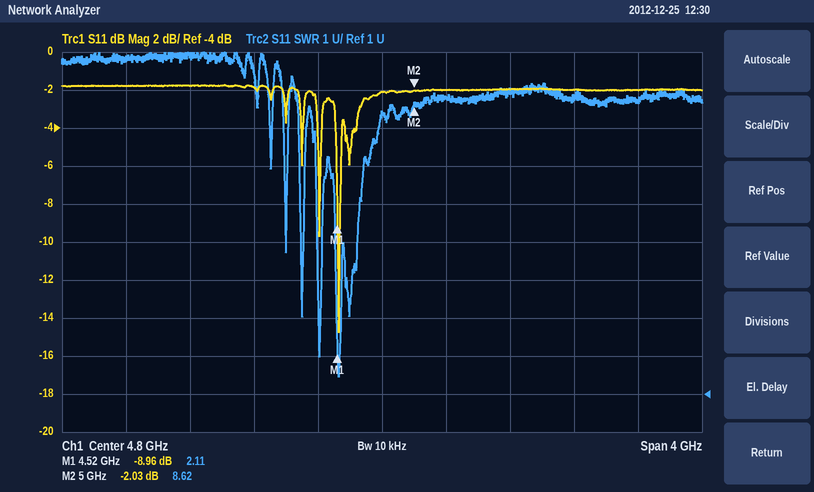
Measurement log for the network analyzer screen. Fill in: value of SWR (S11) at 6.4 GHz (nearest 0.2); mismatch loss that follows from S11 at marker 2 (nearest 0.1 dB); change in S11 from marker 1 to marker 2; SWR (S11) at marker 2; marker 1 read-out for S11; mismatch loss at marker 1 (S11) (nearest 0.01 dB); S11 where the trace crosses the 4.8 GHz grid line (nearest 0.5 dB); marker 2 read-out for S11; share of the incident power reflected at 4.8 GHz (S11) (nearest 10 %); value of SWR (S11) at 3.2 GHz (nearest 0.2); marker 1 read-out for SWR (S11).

8.8
4.3 dB
6.93 dB
8.62
-8.96 dB
0.59 dB
-2.0 dB
-2.03 dB
60 %
9.8
2.11
